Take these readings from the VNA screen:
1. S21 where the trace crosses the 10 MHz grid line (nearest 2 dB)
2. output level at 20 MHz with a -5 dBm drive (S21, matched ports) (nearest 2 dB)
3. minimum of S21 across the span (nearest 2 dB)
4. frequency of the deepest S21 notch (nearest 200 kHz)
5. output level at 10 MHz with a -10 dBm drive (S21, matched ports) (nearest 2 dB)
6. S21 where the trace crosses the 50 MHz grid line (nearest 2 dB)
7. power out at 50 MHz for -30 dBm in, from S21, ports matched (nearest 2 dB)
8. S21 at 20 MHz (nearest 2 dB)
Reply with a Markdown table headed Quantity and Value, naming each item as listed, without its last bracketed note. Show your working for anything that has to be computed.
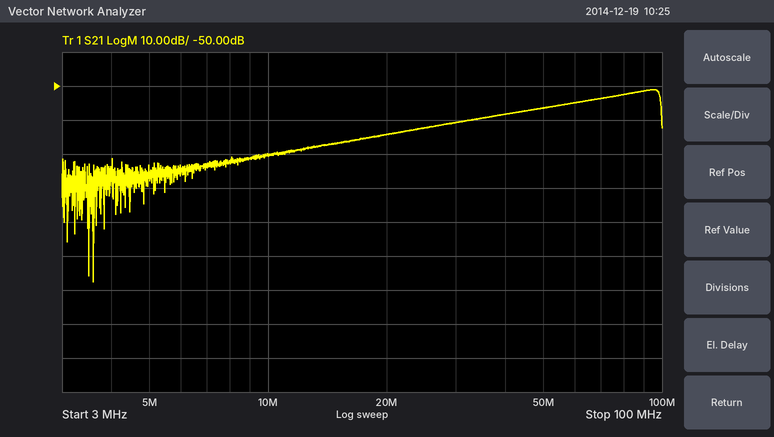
| Quantity | Value |
|---|---|
| S21 where the trace crosses the 10 MHz grid line | -70 dB |
| output level at 20 MHz with a -5 dBm drive (S21, matched ports) | -5 dBm + (-64 dB) = -70 dBm |
| minimum of S21 across the span | -108 dB |
| frequency of the deepest S21 notch | 3.6 MHz |
| output level at 10 MHz with a -10 dBm drive (S21, matched ports) | -10 dBm + (-70 dB) = -80 dBm |
| S21 where the trace crosses the 50 MHz grid line | -56 dB |
| power out at 50 MHz for -30 dBm in, from S21, ports matched | -30 dBm + (-56 dB) = -86 dBm |
| S21 at 20 MHz | -64 dB |
